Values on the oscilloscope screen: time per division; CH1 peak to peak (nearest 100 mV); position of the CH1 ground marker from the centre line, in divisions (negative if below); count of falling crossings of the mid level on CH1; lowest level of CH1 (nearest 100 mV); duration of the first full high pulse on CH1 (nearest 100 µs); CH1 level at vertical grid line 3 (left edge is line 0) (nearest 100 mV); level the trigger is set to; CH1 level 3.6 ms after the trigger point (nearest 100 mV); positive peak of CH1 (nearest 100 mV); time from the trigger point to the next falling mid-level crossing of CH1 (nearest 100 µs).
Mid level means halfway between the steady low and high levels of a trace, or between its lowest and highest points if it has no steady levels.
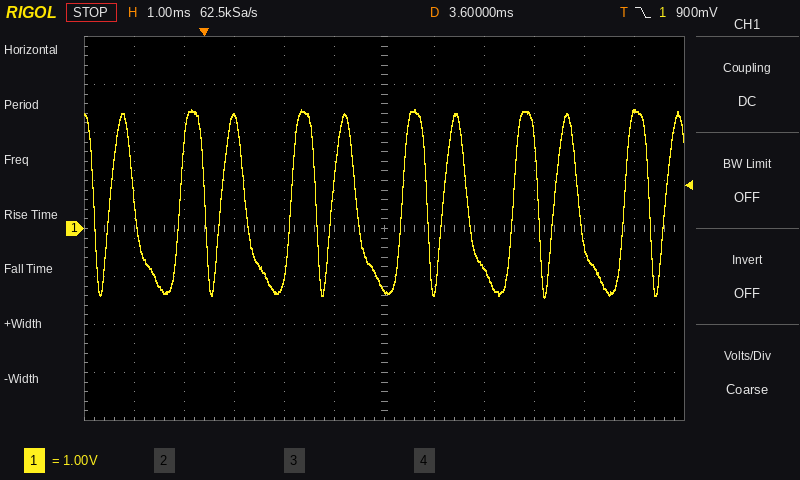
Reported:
1 ms
3.9 V
0.0 div
11
-1.4 V
500 µs
2.3 V
900 mV
-1.3 V
2.5 V
800 µs
